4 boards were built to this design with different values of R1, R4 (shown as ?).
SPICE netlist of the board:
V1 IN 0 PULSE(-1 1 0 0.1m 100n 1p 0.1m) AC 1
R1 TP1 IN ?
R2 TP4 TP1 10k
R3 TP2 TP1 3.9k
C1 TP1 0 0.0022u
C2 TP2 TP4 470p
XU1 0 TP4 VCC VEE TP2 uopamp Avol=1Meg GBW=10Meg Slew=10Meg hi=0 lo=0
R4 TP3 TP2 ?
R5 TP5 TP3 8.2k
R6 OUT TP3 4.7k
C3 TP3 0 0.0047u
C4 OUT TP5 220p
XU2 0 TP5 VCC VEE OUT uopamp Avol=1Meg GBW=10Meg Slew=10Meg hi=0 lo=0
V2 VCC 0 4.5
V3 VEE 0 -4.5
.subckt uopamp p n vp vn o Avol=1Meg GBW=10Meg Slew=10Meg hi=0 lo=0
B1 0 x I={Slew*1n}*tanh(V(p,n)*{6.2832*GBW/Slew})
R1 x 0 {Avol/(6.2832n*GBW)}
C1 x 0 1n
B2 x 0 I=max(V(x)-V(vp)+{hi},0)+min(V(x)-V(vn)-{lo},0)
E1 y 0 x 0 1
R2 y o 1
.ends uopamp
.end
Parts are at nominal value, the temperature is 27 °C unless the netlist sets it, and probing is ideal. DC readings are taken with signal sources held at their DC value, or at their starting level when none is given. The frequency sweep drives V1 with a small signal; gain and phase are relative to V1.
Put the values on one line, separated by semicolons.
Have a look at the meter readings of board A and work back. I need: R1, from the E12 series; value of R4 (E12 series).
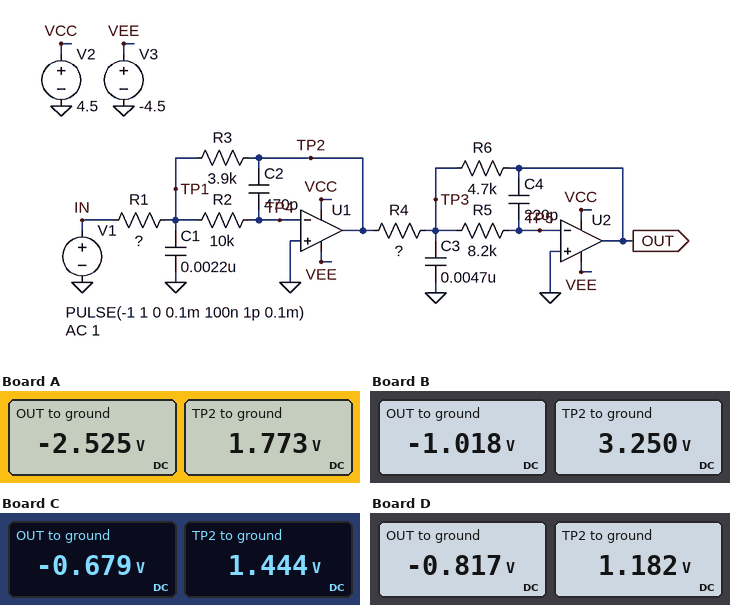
2.2 kΩ; 3.3 kΩ
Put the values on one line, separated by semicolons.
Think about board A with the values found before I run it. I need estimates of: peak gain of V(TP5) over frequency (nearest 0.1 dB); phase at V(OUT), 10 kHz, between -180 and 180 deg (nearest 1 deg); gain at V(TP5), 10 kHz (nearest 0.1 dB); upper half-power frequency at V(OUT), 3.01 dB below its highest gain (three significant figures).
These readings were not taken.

-49.3 dB; -70 deg; -53.1 dB; 18.9 kHz
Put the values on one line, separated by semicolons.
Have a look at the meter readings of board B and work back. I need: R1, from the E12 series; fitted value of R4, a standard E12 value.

1.2 kΩ; 15 kΩ
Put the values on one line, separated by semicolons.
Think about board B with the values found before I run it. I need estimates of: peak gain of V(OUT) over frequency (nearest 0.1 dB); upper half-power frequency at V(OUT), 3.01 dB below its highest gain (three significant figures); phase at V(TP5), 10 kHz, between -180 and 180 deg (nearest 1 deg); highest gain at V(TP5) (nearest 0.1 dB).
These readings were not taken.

0.2 dB; 10.4 kHz; -163 deg; -56.9 dB
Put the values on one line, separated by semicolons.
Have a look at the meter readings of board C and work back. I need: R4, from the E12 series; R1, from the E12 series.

10 kΩ; 2.7 kΩ
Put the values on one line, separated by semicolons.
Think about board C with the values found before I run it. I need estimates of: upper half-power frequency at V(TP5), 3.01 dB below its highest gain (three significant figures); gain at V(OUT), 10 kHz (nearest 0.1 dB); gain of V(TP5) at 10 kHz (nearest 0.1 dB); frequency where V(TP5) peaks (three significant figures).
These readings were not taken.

29.5 kHz; -3.7 dB; -63.7 dB; 23.1 kHz
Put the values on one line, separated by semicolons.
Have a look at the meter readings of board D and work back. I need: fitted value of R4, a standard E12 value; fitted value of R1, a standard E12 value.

6.8 kΩ; 3.3 kΩ
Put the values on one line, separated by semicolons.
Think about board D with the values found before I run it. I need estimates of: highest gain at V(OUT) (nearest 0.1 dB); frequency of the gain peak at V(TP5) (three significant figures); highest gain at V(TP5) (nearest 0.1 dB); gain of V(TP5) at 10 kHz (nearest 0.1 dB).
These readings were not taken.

-1.5 dB; 22.7 kHz; -55.2 dB; -61.7 dB
